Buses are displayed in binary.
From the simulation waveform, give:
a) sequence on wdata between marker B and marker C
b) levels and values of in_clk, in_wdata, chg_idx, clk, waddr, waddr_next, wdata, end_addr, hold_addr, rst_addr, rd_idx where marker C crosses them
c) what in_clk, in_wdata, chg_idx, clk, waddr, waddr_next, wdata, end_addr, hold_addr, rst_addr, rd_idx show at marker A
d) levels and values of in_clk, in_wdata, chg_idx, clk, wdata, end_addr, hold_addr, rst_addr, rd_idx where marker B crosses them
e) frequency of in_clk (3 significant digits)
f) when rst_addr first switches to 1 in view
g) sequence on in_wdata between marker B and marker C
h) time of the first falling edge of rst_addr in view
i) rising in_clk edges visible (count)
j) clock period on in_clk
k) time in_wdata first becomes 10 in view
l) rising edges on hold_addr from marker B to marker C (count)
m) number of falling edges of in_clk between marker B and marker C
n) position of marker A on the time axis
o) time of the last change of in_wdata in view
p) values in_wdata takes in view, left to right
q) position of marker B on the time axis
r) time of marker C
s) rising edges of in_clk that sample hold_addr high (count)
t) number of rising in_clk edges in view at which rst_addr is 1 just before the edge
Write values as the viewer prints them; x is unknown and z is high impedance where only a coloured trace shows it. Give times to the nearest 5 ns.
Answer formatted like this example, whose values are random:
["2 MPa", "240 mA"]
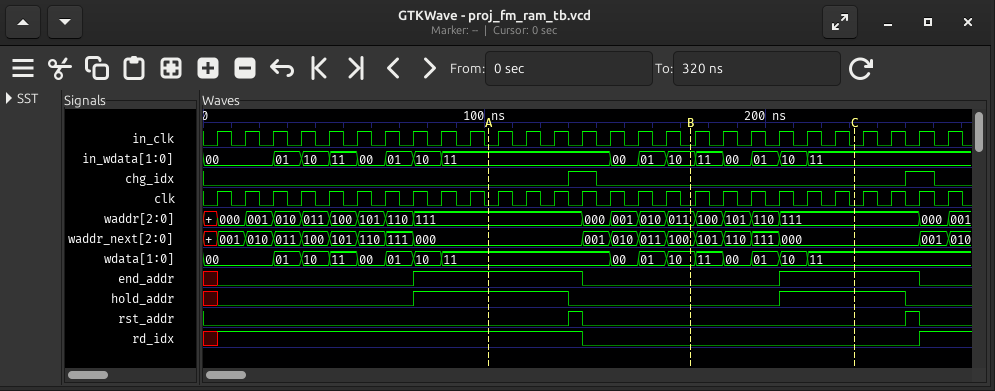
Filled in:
["10, 11, 00, 01, 10, 11", "in_clk=0, in_wdata=11, chg_idx=0, clk=0, waddr=111, waddr_next=000, wdata=11, end_addr=1, hold_addr=1, rst_addr=0, rd_idx=0", "in_clk=0, in_wdata=11, chg_idx=0, clk=0, waddr=111, waddr_next=000, wdata=11, end_addr=1, hold_addr=1, rst_addr=0, rd_idx=1", "in_clk=0, in_wdata=10, chg_idx=0, clk=0, wdata=10, end_addr=0, hold_addr=0, rst_addr=0, rd_idx=0", "100 MHz", "130 ns", "10, 11, 00, 01, 10, 11", "135 ns", "27", "10 ns", "35 ns", "1", "6", "100 ns", "215 ns", "00, 01, 10, 11, 00, 01, 10, 11, 00, 01, 10, 11, 00, 01, 10, 11", "175 ns", "230 ns", "9", "2"]
